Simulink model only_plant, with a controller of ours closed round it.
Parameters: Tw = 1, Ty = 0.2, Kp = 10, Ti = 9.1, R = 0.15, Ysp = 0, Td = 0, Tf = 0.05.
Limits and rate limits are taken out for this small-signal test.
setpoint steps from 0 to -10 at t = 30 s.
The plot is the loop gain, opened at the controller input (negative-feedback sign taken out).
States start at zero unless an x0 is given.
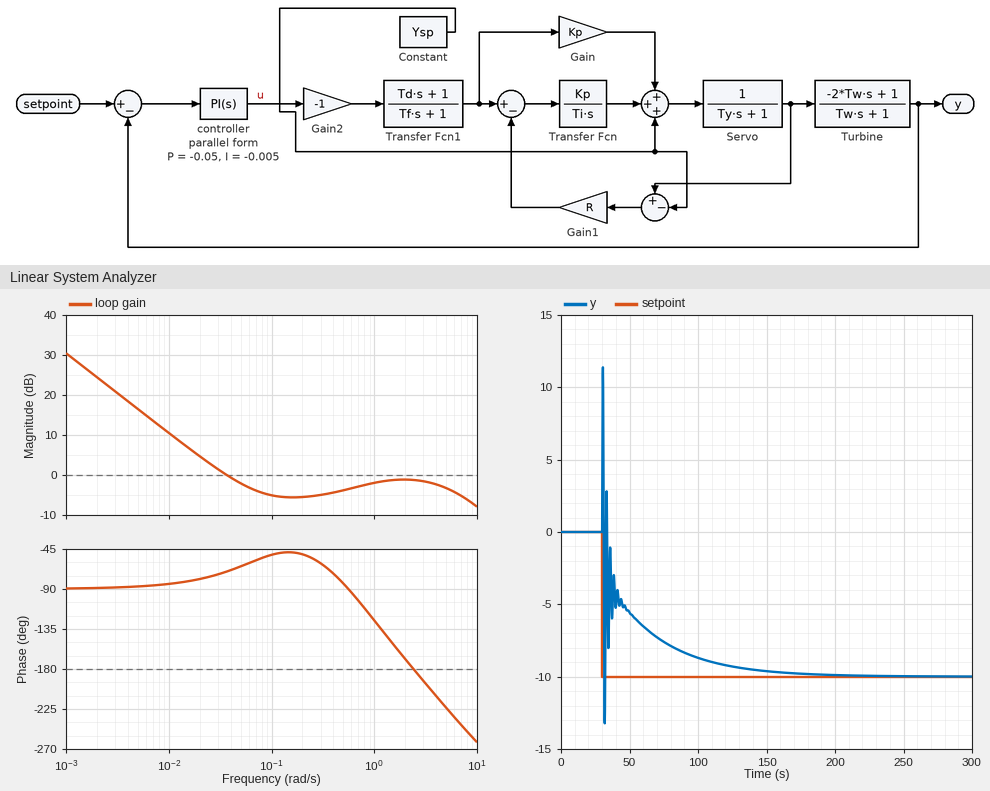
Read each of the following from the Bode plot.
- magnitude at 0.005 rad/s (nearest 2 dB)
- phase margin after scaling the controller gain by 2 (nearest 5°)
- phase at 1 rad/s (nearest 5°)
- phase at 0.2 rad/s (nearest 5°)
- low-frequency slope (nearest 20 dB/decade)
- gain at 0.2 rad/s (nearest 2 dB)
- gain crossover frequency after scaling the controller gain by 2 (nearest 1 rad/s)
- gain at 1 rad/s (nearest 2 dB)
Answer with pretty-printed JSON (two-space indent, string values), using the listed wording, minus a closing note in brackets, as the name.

{
  "magnitude at 0.005 rad/s": "16 dB",
  "phase margin after scaling the controller gain by 2": "-70°",
  "phase at 1 rad/s": "-125°",
  "phase at 0.2 rad/s": "-50°",
  "low-frequency slope": "-20 dB/decade",
  "gain at 0.2 rad/s": "-6 dB",
  "gain crossover frequency after scaling the controller gain by 2": "8 rad/s",
  "gain at 1 rad/s": "-2 dB"
}
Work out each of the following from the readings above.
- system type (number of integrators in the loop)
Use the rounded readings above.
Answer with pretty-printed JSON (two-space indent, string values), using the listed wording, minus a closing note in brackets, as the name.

{
  "system type": "1"
}
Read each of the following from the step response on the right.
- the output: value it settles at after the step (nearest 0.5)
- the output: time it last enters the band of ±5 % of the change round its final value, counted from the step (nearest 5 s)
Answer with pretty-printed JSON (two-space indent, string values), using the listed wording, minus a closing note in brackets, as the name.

{
  "the output: value it settles at after the step": "-10.0",
  "the output: time it last enters the band of ±5 % of the change round its final value, counted from the step": "110 s"
}
